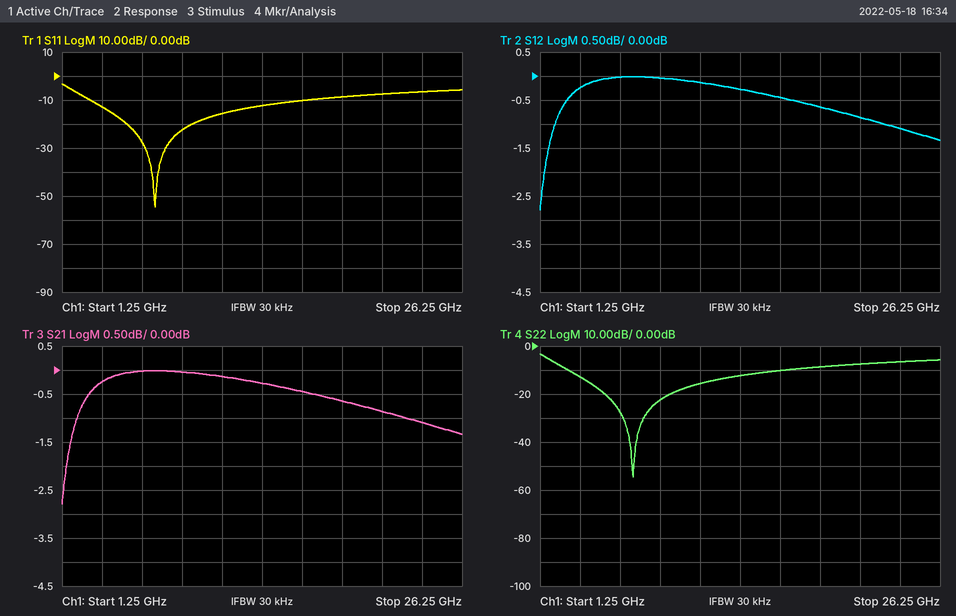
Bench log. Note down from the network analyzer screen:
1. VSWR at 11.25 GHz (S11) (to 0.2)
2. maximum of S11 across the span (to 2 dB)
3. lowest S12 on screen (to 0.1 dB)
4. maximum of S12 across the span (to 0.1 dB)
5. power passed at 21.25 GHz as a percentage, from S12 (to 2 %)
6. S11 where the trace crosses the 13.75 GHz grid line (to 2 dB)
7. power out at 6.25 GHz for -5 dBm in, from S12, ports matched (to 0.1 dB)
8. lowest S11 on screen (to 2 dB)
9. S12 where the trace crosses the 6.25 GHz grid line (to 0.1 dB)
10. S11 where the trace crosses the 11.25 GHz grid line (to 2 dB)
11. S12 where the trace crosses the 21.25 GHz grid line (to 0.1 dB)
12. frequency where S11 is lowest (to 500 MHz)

1.4
-4 dB
-2.8 dB
0.0 dB
82 %
-12 dB
-5.0 dBm
-54 dB
0.0 dB
-16 dB
-0.9 dB
7.0 GHz
